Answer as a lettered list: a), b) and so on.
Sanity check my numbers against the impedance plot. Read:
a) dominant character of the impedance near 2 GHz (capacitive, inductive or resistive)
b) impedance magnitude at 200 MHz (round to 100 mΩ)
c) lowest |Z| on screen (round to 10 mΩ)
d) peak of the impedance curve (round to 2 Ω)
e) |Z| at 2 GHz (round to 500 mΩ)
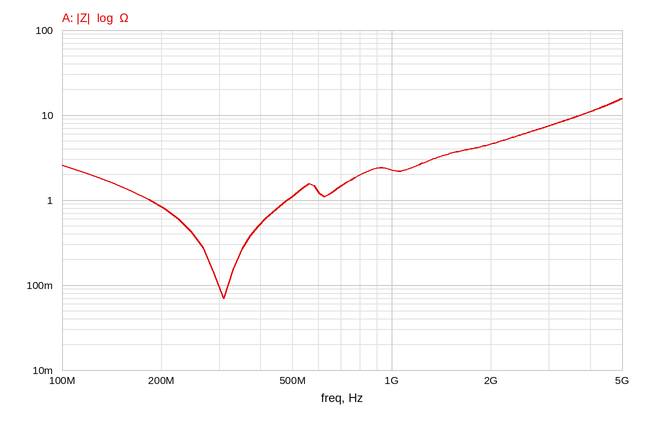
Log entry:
a) inductive
b) 800 mΩ
c) 70 mΩ
d) 16 Ω
e) 4.5 Ω
